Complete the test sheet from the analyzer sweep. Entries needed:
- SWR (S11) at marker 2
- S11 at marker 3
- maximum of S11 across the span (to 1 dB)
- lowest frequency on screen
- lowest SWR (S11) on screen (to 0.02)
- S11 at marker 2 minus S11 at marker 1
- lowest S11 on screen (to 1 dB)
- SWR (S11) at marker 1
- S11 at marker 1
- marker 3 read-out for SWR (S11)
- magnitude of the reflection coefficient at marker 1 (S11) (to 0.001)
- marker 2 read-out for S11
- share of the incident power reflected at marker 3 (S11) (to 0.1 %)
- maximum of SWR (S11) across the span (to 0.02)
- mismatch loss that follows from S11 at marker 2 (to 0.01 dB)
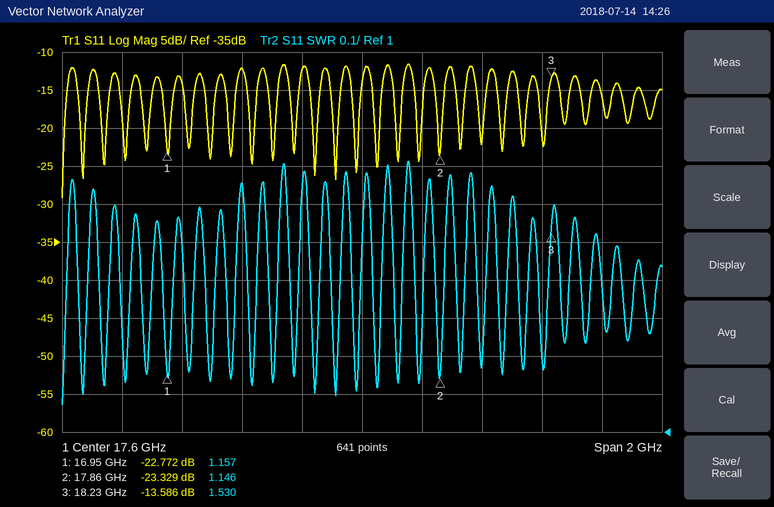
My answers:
1.146
-13.586 dB
-12 dB
16.6 GHz
1.08
-0.557 dB
-29 dB
1.157
-22.772 dB
1.530
0.073
-23.329 dB
4.4 %
1.72
0.02 dB
